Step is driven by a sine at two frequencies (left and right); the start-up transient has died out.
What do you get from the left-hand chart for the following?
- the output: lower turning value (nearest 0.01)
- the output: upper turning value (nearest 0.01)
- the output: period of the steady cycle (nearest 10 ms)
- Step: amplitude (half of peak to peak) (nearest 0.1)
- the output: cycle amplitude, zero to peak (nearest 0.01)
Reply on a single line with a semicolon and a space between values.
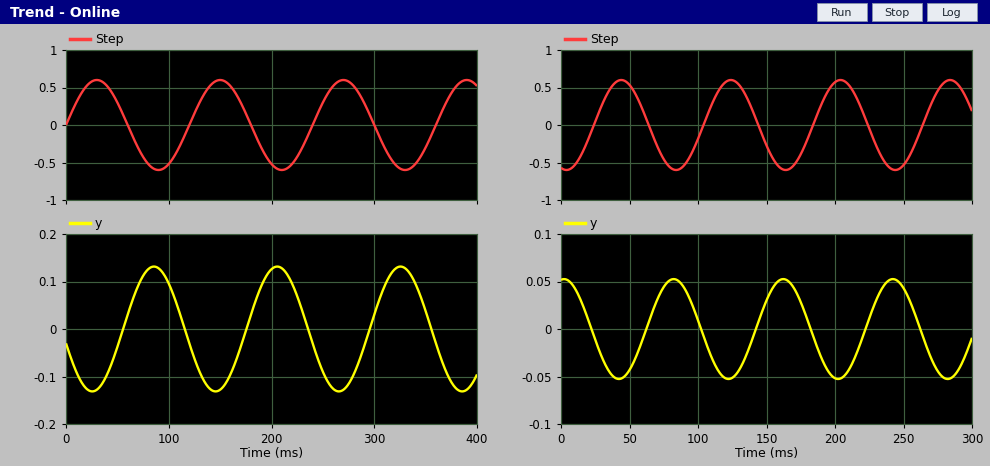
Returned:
-0.13; 0.13; 120 ms; 0.6; 0.13
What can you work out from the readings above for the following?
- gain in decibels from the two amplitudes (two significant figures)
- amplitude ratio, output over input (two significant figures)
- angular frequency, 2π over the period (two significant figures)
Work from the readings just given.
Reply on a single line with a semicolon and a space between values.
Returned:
-13 dB; 0.22; 0.052 rad/ms
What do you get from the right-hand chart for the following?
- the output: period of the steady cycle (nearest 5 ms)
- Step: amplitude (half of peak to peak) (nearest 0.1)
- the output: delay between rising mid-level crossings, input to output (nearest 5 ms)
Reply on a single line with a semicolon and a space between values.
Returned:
80 ms; 0.6; 40 ms
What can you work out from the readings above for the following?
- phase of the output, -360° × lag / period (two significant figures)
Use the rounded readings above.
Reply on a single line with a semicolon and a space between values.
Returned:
-180°
